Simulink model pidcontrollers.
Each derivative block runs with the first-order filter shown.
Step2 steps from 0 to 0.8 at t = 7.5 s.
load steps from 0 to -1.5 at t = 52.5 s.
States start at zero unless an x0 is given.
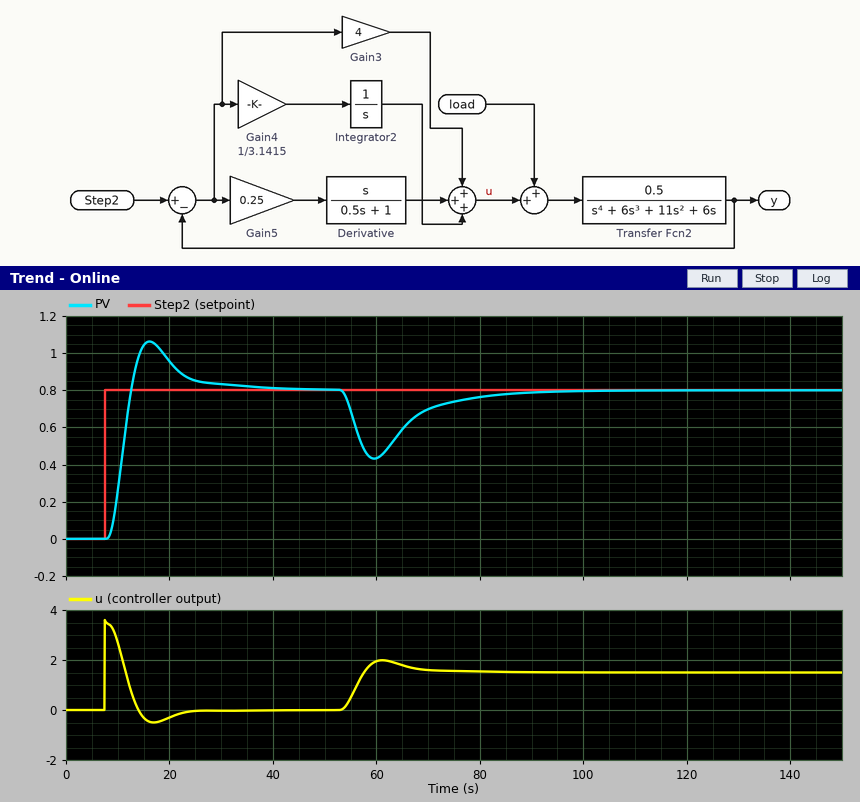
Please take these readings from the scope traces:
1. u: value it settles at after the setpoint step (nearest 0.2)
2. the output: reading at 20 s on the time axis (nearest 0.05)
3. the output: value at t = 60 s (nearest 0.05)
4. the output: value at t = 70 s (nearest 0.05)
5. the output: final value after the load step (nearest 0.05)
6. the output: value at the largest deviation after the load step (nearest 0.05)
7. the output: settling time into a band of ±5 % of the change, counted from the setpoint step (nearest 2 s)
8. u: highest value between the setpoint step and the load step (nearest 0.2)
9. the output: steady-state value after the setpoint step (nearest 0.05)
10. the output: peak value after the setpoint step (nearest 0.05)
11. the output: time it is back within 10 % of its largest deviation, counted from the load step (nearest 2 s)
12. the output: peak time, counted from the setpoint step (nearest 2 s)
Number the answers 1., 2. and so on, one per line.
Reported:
1. 0.0
2. 0.95
3. 0.45
4. 0.70
5. 0.80
6. 0.45
7. 20 s
8. 3.6
9. 0.80
10. 1.05
11. 28 s
12. 8 s
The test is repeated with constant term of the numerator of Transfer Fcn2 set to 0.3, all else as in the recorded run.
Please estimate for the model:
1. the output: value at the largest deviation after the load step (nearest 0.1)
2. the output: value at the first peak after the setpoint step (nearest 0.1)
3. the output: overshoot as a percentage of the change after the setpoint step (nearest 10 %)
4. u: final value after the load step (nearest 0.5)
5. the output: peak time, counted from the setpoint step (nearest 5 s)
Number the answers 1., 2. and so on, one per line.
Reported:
1. 0.5
2. 1.0
3. 30 %
4. 1.5
5. 15 s
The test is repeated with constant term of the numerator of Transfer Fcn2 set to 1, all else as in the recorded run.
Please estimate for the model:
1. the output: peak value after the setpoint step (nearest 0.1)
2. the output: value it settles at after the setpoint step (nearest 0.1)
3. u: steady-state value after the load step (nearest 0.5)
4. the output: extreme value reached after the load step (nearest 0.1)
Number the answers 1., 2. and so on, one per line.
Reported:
1. 1.2
2. 0.8
3. 1.5
4. 0.3
